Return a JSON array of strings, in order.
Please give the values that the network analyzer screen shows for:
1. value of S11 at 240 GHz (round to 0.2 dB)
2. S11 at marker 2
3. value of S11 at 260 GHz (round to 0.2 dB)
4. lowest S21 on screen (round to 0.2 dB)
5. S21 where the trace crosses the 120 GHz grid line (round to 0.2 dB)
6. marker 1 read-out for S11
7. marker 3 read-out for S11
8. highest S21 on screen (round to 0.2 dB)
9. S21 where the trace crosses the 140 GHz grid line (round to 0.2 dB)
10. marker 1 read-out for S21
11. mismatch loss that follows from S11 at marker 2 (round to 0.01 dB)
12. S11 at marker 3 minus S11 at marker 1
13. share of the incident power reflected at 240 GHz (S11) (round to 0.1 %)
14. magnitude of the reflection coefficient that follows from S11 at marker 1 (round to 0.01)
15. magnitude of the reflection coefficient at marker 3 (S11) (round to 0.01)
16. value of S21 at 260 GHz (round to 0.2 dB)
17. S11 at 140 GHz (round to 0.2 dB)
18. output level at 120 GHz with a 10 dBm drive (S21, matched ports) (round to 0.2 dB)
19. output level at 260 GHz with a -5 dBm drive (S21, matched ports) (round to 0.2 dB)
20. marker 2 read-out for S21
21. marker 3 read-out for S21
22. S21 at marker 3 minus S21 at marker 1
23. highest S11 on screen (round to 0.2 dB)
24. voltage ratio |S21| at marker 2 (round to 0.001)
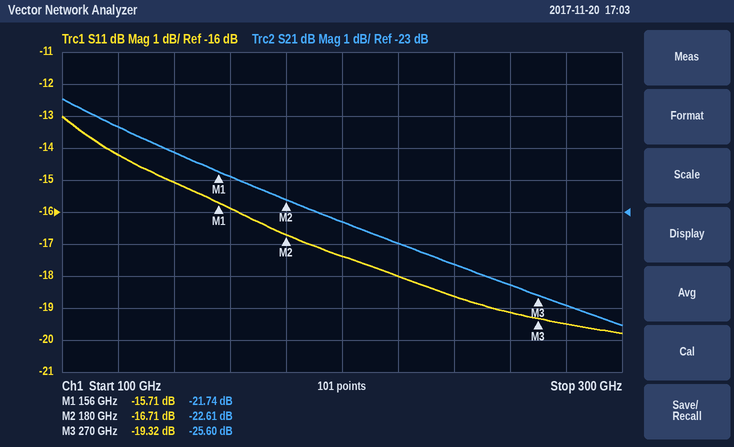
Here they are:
["-18.6 dB", "-16.71 dB", "-19.2 dB", "-26.6 dB", "-20.4 dB", "-15.71 dB", "-19.32 dB", "-19.4 dB", "-21.2 dB", "-21.74 dB", "0.09 dB", "-3.61 dB", "1.4 %", "0.16", "0.11", "-25.2 dB", "-15.0 dB", "-10.4 dBm", "-30.2 dBm", "-22.61 dB", "-25.60 dB", "-3.86 dB", "-13.0 dB", "0.074"]
